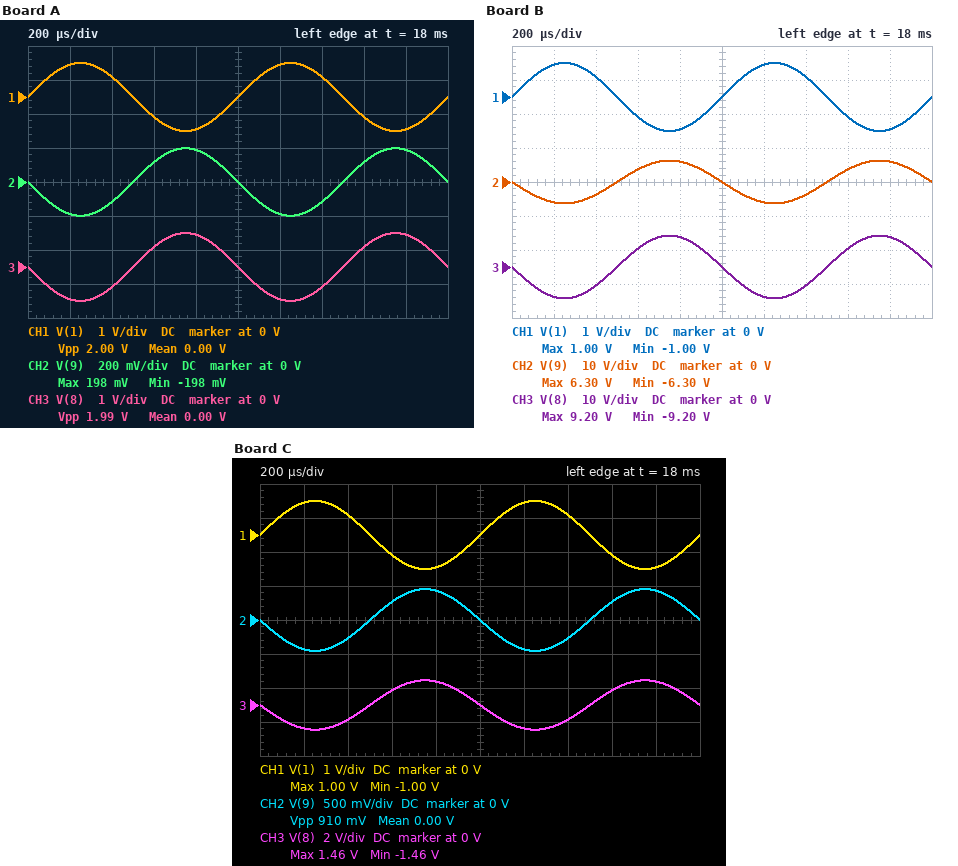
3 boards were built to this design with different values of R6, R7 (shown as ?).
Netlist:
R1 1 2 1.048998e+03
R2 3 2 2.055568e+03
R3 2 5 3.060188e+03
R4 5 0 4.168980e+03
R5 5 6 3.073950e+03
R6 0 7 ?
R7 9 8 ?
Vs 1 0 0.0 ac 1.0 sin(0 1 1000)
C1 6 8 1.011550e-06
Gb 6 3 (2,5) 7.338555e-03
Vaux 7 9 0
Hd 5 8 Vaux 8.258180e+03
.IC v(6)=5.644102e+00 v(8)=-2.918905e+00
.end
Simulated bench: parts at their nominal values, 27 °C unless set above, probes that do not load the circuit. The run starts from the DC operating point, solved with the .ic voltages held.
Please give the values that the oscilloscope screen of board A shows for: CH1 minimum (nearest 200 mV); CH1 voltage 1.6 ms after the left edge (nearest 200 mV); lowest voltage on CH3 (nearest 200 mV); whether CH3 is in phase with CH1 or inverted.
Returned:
-1.0 V
-600 mV
-1.0 V
inverted
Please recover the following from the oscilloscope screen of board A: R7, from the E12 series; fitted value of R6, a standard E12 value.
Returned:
3.3 kΩ
820 Ω
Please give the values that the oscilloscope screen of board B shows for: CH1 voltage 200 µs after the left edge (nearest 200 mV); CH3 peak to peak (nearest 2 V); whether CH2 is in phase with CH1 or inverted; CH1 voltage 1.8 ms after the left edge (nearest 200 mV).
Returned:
1.0 V
18 V
inverted
-1.0 V
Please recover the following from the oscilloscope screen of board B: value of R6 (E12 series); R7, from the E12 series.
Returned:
4.7 kΩ
2.2 kΩ
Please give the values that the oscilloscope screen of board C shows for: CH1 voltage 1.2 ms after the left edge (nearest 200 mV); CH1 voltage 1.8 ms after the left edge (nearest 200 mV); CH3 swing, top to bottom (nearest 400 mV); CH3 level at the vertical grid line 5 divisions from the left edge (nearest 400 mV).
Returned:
1.0 V
-1.0 V
2.8 V
0 V
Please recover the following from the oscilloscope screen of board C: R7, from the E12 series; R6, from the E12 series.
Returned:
3.3 kΩ
1.5 kΩ
